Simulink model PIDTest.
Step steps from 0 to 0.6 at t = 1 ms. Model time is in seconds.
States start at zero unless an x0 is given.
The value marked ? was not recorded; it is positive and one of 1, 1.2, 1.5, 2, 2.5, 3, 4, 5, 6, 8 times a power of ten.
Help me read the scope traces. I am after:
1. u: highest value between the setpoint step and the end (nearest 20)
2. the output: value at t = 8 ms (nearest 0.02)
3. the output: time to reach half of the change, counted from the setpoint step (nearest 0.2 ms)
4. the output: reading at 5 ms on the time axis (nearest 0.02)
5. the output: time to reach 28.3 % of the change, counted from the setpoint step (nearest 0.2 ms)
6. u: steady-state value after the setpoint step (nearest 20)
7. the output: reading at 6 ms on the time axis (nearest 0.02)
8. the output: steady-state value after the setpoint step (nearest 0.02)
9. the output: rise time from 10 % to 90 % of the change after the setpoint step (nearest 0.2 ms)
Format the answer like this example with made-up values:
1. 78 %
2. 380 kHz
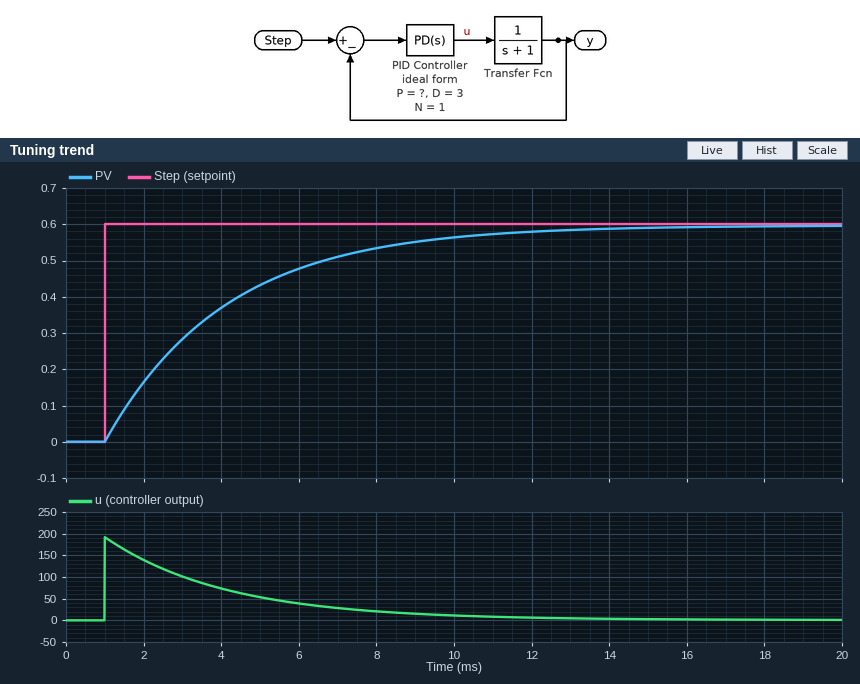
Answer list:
1. 200
2. 0.54
3. 2.2 ms
4. 0.44
5. 1.0 ms
6. 0
7. 0.48
8. 0.60
9. 6.8 ms
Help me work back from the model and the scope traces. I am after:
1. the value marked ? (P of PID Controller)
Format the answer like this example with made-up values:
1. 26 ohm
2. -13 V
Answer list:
1. 80
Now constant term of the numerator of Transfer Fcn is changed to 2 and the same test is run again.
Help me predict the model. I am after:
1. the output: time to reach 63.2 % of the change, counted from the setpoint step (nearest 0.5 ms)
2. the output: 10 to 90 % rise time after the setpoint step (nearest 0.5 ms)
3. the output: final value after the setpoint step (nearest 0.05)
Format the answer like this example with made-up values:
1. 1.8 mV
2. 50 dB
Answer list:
1. 1.5 ms
2. 3.5 ms
3. 0.60
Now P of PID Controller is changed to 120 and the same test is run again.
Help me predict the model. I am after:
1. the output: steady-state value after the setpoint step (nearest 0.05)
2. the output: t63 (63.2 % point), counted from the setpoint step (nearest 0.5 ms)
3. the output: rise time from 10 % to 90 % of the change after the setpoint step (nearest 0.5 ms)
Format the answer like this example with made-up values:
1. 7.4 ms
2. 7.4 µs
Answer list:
1. 0.60
2. 2.0 ms
3. 4.5 ms
